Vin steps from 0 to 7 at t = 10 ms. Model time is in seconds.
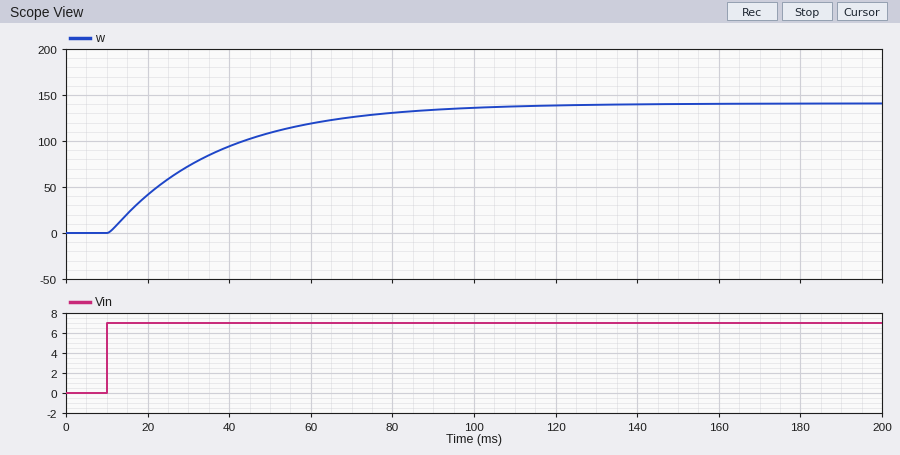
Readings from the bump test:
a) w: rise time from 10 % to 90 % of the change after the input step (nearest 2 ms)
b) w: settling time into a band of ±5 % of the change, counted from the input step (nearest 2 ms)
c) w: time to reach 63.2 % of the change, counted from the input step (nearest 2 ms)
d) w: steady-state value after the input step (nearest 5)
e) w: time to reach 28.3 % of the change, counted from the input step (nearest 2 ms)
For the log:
58 ms
80 ms
28 ms
140
10 ms
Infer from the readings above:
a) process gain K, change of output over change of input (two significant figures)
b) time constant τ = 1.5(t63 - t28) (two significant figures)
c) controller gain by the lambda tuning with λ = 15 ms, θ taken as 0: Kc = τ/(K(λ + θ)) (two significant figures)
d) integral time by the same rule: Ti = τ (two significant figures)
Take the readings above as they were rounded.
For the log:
20
27 ms
0.090
27 ms
